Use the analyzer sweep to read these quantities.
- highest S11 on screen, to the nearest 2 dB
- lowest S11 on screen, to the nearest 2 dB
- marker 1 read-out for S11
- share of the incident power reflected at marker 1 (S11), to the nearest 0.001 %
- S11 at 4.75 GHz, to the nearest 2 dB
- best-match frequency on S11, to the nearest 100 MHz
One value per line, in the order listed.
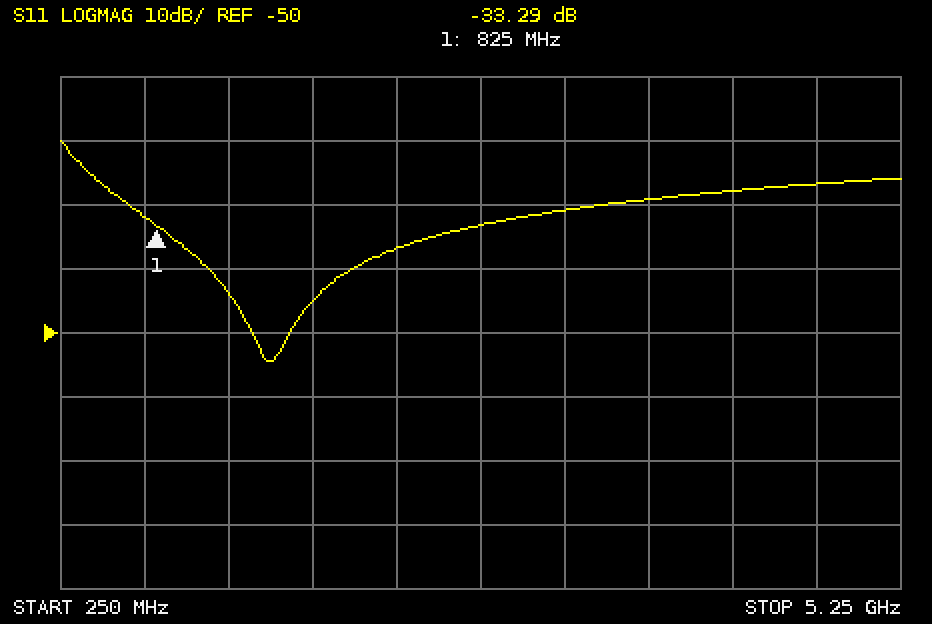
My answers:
-20 dB
-54 dB
-33.29 dB
0.047 %
-26 dB
1.5 GHz
